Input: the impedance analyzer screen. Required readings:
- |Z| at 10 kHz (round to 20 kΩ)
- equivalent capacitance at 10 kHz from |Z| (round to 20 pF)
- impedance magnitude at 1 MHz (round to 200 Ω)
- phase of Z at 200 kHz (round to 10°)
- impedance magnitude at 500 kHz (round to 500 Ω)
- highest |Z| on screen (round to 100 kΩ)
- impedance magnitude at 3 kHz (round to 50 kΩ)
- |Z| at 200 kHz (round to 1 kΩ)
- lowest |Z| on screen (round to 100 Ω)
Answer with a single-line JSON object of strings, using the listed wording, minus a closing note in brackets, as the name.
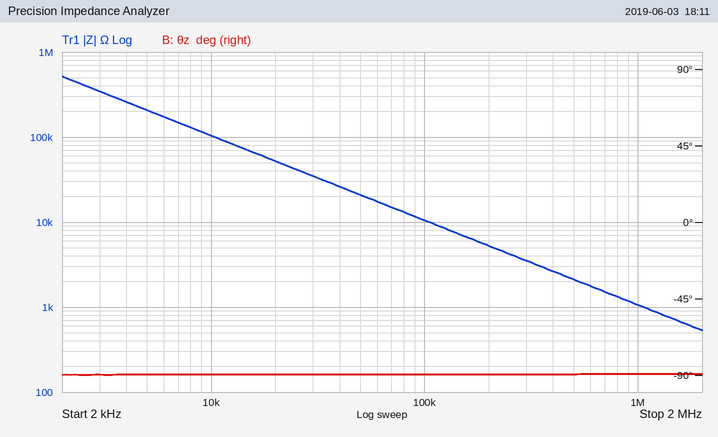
{"|Z| at 10 kHz": "100 kΩ", "equivalent capacitance at 10 kHz from |Z|": "160 pF", "impedance magnitude at 1 MHz": "1.0 kΩ", "phase of Z at 200 kHz": "-90°", "impedance magnitude at 500 kHz": "2.0 kΩ", "highest |Z| on screen": "500 kΩ", "impedance magnitude at 3 kHz": "350 kΩ", "|Z| at 200 kHz": "5 kΩ", "lowest |Z| on screen": "500 Ω"}
